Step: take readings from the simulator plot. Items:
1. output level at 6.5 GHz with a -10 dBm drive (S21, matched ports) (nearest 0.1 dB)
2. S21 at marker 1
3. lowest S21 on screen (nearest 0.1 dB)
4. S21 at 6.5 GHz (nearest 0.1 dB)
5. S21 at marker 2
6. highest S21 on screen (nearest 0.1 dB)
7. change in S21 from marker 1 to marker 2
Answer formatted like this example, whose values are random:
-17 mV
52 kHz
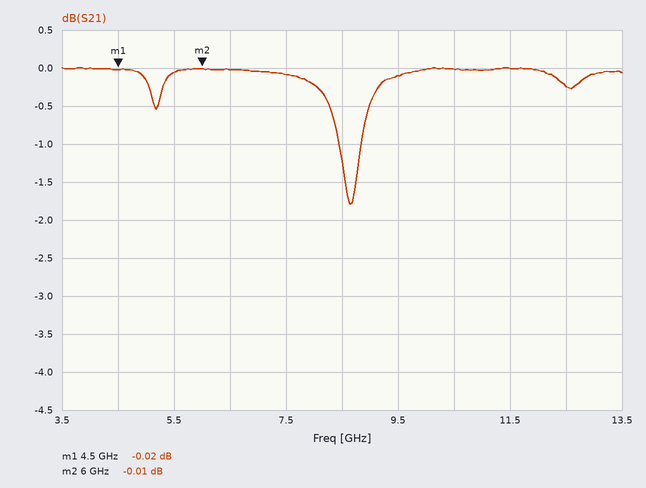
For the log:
-10.0 dBm
-0.02 dB
-1.8 dB
0.0 dB
-0.01 dB
0.0 dB
0.01 dB
